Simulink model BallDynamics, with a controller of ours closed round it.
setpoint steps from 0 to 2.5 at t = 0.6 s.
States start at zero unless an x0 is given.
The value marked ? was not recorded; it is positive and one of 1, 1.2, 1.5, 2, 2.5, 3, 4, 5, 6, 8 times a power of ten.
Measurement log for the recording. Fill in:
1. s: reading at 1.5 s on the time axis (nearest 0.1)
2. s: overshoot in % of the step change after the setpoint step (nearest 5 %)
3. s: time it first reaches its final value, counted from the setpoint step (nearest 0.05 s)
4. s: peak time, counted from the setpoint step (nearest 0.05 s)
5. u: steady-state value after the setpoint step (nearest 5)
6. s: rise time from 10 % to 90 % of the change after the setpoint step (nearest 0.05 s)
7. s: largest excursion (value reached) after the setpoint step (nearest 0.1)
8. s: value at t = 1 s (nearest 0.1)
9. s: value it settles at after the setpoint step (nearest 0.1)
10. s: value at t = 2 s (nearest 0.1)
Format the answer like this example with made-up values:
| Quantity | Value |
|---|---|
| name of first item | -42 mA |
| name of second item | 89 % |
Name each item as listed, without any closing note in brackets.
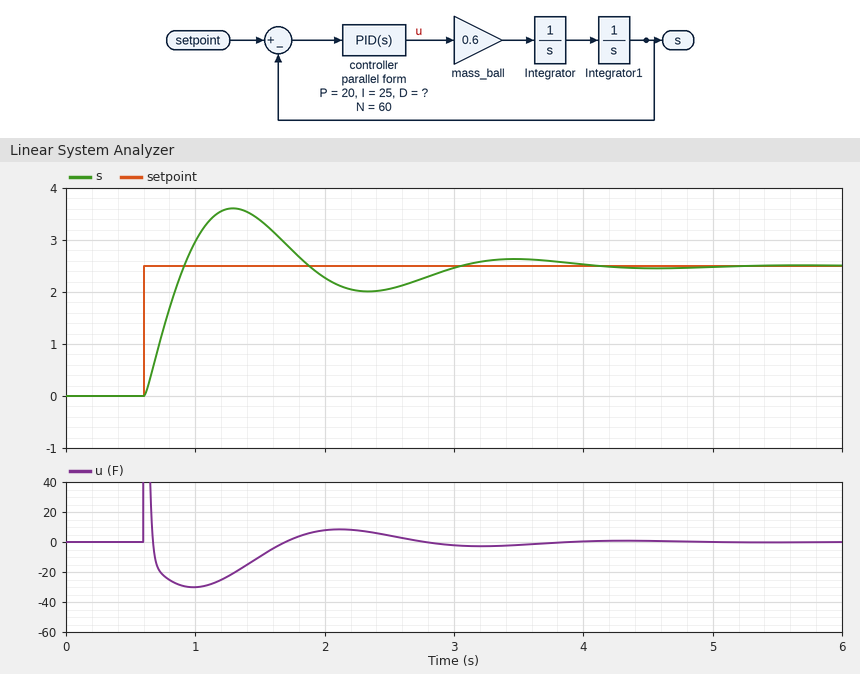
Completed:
| Quantity | Value |
|---|---|
| s: reading at 1.5 s on the time axis | 3.4 |
| s: overshoot in % of the step change after the setpoint step | 45 % |
| s: time it first reaches its final value, counted from the setpoint step | 0.30 s |
| s: peak time, counted from the setpoint step | 0.70 s |
| u: steady-state value after the setpoint step | 0 |
| s: rise time from 10 % to 90 % of the change after the setpoint step | 0.25 s |
| s: largest excursion (value reached) after the setpoint step | 3.6 |
| s: value at t = 1 s | 3.0 |
| s: value it settles at after the setpoint step | 2.5 |
| s: value at t = 2 s | 2.3 |
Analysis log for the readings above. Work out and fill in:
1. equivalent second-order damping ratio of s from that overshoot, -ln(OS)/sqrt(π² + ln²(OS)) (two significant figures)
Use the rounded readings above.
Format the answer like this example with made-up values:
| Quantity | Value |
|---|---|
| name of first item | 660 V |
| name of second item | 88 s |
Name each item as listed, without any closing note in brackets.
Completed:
| Quantity | Value |
|---|---|
| equivalent second-order damping ratio of s from that overshoot, -ln(OS)/sqrt(π² + ln²(OS)) | 0.25 |
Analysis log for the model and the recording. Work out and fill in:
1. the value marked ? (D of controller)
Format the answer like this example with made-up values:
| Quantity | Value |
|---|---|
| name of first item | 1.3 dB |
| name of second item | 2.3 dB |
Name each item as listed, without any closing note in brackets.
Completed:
| Quantity | Value |
|---|---|
| the value marked ? | 6 |
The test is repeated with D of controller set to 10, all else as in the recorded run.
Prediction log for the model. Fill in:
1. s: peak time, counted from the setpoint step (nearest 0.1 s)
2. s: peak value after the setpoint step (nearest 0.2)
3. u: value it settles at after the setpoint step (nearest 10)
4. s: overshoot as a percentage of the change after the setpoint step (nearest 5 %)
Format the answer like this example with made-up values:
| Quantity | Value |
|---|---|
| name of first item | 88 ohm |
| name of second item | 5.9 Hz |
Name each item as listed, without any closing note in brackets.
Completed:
| Quantity | Value |
|---|---|
| s: peak time, counted from the setpoint step | 0.6 s |
| s: peak value after the setpoint step | 3.2 |
| u: value it settles at after the setpoint step | 0 |
| s: overshoot as a percentage of the change after the setpoint step | 25 % |
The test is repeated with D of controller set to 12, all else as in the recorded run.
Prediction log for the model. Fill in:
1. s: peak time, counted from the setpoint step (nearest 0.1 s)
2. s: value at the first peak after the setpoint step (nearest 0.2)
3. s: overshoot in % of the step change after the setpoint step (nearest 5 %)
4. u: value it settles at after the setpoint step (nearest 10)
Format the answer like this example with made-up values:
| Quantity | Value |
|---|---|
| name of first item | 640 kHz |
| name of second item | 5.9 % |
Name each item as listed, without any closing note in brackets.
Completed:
| Quantity | Value |
|---|---|
| s: peak time, counted from the setpoint step | 0.6 s |
| s: value at the first peak after the setpoint step | 3.0 |
| s: overshoot in % of the step change after the setpoint step | 20 % |
| u: value it settles at after the setpoint step | 0 |
